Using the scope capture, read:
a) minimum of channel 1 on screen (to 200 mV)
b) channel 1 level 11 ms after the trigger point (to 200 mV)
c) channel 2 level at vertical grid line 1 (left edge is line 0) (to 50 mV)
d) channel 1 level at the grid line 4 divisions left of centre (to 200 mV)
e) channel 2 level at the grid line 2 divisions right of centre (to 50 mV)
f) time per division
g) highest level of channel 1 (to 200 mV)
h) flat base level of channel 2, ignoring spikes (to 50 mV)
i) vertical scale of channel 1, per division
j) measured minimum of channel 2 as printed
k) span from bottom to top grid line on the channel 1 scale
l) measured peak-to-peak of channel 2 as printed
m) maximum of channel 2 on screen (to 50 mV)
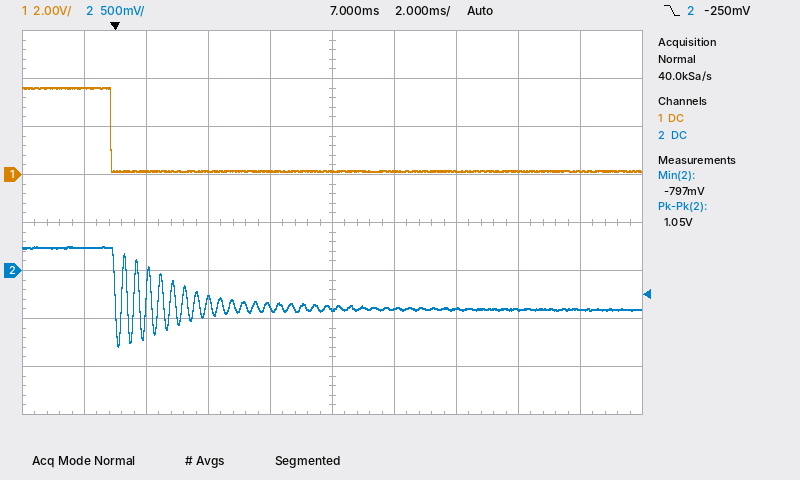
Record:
200 mV
200 mV
250 mV
3.6 V
-400 mV
2 ms
3.6 V
-400 mV
2 V
-797 mV
16 V
1.05 V
250 mV
